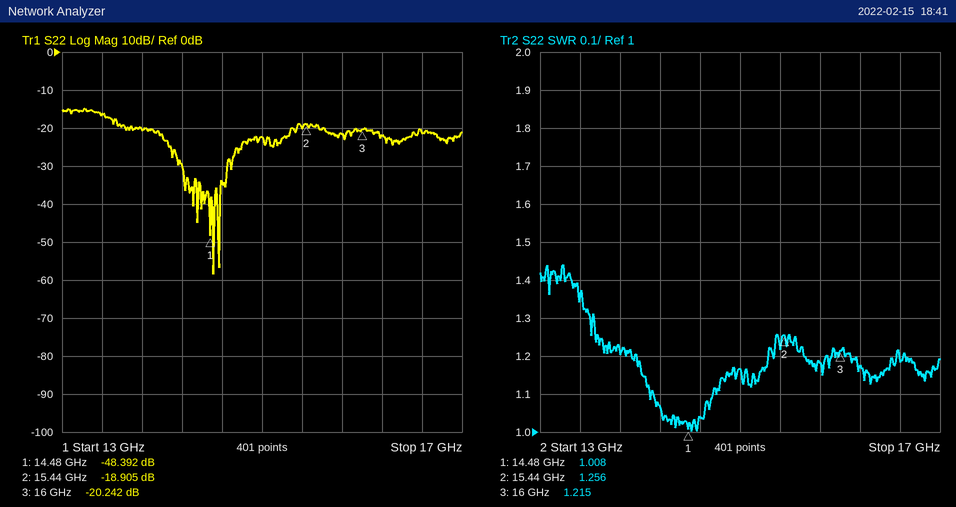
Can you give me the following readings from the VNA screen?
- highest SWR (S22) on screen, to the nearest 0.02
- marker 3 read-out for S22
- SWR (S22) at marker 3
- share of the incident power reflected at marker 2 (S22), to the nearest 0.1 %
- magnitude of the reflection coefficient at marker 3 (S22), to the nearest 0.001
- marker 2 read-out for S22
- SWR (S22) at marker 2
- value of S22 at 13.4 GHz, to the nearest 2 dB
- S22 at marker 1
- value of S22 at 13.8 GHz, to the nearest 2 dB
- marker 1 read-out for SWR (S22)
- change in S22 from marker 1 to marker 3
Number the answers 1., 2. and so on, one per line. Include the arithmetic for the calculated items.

1. 1.44
2. -20.242 dB
3. 1.215
4. 10^(-18.905/10) ≈ 1.3 %
5. 10^(-20.242/20) ≈ 0.097
6. -18.905 dB
7. 1.256
8. -16 dB
9. -48.392 dB
10. -20 dB
11. 1.008
12. -20.242 − (-48.392) = 28.150 dB
